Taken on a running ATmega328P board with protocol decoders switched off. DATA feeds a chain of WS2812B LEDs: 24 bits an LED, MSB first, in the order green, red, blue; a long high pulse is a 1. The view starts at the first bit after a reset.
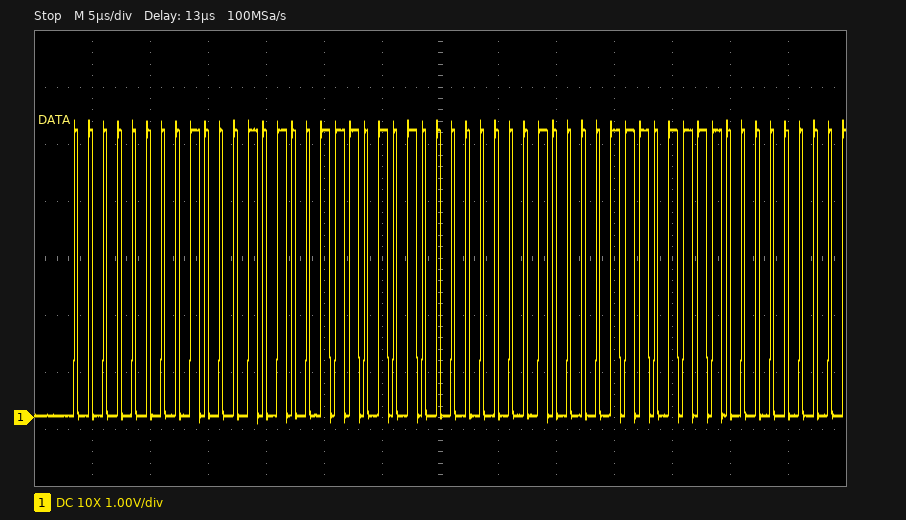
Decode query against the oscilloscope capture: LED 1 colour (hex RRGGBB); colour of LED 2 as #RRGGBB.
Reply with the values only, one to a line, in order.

#8A0075
#870078
